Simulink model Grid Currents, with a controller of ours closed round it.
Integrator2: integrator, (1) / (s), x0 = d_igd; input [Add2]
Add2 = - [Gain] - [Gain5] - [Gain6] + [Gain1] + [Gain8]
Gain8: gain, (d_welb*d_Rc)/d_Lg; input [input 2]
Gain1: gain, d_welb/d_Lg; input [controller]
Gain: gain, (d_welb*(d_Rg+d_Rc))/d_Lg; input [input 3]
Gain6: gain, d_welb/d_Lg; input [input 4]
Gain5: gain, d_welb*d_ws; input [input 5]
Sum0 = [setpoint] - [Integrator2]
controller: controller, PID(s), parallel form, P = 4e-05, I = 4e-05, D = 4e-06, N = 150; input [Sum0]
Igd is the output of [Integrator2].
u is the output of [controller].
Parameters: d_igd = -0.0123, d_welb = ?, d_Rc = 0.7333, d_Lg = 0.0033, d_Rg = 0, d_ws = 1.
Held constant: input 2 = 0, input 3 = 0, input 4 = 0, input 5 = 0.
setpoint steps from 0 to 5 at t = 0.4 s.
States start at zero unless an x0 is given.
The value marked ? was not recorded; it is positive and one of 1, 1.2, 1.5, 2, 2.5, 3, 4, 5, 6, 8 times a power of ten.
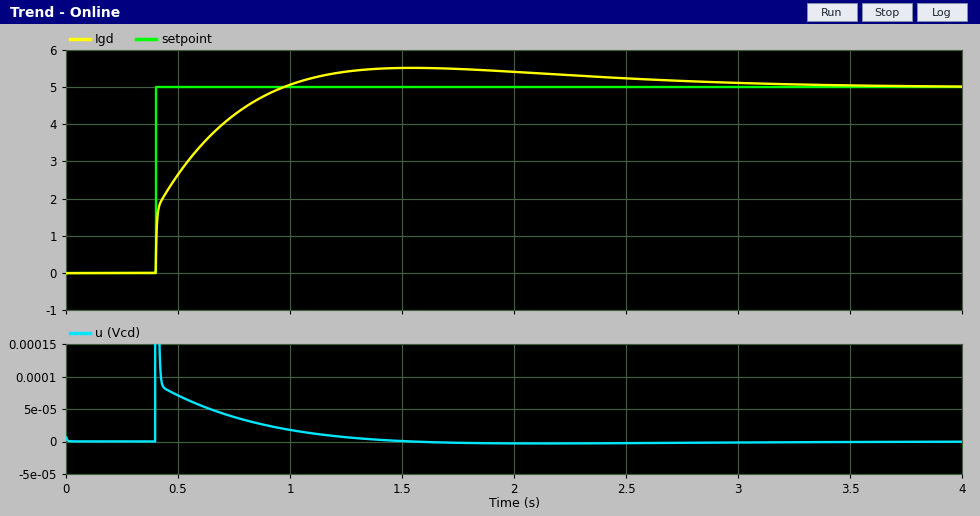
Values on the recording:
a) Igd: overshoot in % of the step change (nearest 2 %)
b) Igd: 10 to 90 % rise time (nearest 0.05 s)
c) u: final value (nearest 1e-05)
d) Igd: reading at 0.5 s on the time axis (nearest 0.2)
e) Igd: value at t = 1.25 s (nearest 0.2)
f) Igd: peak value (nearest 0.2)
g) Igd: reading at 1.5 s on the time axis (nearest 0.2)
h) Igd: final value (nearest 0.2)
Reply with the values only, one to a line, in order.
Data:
10 %
0.40 s
0.00000
2.6
5.4
5.6
5.6
5.0
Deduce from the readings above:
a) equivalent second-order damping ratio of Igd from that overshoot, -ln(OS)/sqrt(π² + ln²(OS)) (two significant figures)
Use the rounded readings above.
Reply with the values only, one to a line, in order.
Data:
0.59
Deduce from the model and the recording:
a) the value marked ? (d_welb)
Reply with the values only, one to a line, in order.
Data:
400
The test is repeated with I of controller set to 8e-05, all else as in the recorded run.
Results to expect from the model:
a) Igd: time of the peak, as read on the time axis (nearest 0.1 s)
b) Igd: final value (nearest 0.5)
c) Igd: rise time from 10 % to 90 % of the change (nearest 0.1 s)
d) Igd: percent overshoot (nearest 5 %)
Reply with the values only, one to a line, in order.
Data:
1.3 s
5.0
0.3 s
15 %
